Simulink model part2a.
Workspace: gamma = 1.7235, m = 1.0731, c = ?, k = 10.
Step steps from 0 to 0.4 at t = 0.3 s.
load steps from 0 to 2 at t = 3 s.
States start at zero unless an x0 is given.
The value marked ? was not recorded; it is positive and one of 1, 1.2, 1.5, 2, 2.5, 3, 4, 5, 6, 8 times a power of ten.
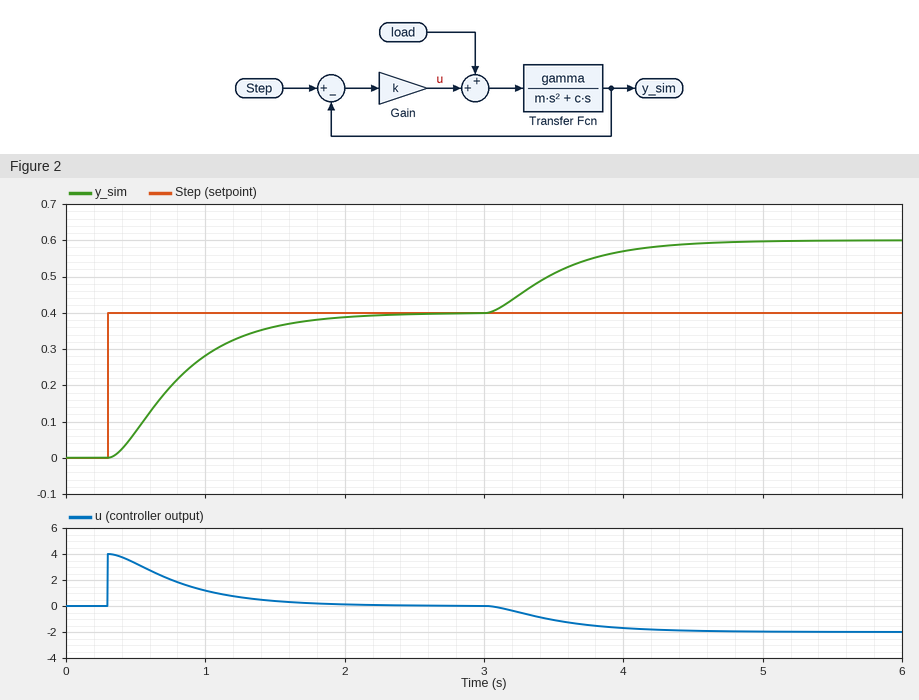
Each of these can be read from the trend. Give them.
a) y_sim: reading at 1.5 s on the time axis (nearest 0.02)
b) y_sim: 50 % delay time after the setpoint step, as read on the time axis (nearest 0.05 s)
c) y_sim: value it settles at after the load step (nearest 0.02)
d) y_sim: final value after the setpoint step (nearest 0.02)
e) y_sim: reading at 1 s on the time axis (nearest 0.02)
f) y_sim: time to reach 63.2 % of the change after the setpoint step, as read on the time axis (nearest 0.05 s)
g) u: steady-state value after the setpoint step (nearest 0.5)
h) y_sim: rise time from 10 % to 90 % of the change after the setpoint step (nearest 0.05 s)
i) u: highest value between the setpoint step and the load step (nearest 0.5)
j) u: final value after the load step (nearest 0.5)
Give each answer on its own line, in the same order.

0.36
0.75 s
0.60
0.40
0.28
0.90 s
0.0
1.05 s
4.0
-2.0
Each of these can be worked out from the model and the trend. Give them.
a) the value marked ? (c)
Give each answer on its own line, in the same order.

10
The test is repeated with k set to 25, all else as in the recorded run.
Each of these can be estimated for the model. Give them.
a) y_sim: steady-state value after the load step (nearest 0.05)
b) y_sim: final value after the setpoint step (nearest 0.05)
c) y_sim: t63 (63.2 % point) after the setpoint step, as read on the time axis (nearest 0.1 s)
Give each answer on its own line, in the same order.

0.50
0.40
0.6 s
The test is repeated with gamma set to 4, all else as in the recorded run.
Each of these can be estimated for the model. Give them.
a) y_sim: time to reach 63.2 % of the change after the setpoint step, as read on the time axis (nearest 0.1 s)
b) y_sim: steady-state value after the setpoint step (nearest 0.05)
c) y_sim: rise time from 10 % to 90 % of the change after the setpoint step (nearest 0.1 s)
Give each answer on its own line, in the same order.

0.6 s
0.40
0.4 s
